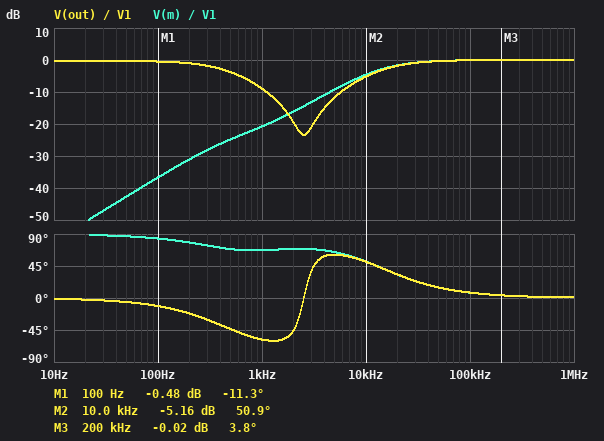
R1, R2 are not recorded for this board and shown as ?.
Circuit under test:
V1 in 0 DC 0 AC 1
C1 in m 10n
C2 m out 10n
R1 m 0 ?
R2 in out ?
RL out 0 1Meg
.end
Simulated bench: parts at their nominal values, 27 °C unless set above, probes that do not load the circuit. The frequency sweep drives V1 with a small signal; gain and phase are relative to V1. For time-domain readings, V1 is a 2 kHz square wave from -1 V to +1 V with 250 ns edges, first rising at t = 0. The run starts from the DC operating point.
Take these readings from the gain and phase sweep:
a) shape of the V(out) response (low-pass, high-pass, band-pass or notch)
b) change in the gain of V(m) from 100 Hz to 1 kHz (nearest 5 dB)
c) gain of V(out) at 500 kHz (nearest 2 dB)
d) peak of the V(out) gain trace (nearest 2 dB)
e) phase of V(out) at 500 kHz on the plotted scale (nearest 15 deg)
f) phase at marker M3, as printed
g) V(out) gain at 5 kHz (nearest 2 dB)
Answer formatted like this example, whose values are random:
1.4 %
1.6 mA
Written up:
notch
15 dB
0 dB
0 dB
0 deg
3.8 deg
-12 dB
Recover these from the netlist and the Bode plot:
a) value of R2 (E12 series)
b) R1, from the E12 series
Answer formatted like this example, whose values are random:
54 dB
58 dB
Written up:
33 kΩ
1.2 kΩ
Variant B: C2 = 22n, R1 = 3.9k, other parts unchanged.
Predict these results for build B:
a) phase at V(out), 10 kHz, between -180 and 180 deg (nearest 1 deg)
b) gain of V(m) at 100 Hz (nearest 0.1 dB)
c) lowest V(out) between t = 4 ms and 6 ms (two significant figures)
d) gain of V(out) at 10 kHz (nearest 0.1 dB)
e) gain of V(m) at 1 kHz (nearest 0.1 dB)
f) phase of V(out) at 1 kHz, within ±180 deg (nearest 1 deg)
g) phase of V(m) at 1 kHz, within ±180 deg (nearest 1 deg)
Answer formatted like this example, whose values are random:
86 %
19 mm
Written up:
22 deg
-23.2 dB
-1.8 V
-0.9 dB
-11.9 dB
8 deg
54 deg
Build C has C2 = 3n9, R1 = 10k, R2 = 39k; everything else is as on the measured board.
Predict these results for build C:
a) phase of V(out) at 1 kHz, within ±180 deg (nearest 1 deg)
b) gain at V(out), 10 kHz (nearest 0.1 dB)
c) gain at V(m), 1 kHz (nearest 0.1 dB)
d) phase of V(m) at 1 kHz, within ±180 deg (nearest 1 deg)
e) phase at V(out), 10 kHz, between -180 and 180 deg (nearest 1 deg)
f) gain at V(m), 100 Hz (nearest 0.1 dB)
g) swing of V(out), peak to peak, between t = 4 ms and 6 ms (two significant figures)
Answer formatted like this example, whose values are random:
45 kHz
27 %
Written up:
-11 deg
-0.3 dB
-5.0 dB
47 deg
9 deg
-21.3 dB
2.9 V
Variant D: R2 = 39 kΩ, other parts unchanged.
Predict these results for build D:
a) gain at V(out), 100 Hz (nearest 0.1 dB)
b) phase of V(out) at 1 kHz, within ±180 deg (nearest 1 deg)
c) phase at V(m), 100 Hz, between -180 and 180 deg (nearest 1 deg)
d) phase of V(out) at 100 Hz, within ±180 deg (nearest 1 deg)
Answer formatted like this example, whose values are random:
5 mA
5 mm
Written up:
-0.6 dB
-61 deg
83 deg
-13 deg
